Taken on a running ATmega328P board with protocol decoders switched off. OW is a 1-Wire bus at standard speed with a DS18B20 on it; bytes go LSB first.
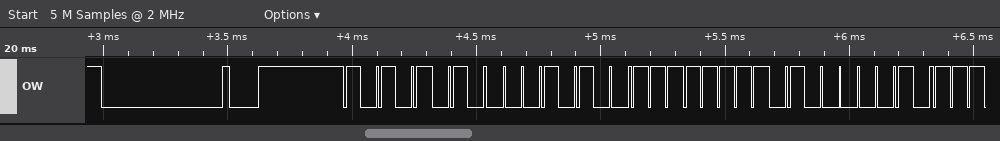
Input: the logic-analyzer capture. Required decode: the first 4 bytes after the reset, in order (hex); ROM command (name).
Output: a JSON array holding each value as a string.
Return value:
["55 28 FF 82", "Match ROM"]
